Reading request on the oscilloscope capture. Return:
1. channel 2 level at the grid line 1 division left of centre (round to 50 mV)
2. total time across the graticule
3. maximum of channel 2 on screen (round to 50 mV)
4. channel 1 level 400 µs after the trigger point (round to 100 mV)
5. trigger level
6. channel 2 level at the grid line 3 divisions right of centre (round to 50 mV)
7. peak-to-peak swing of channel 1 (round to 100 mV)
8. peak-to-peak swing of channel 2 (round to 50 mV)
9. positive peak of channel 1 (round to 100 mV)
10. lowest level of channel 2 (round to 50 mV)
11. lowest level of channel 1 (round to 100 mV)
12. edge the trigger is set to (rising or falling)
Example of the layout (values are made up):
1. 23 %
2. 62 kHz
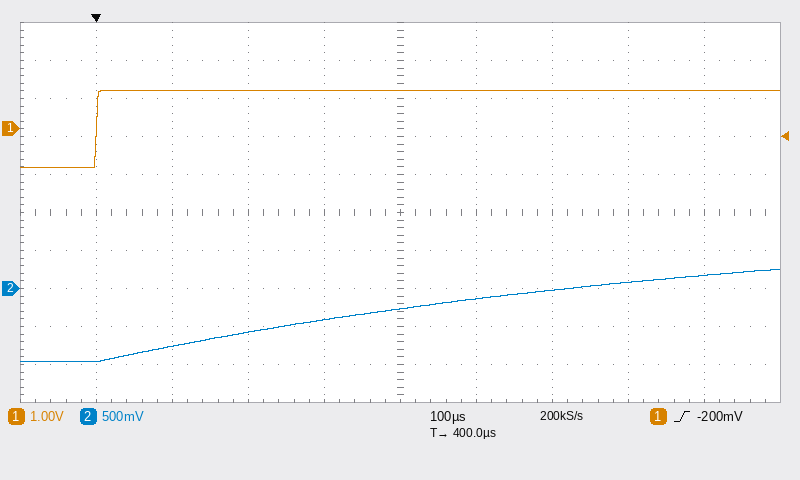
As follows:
1. -400 mV
2. 1 ms
3. 250 mV
4. 1.0 V
5. -200 mV
6. 100 mV
7. 2.0 V
8. 1.20 V
9. 1.0 V
10. -950 mV
11. -1.0 V
12. rising
